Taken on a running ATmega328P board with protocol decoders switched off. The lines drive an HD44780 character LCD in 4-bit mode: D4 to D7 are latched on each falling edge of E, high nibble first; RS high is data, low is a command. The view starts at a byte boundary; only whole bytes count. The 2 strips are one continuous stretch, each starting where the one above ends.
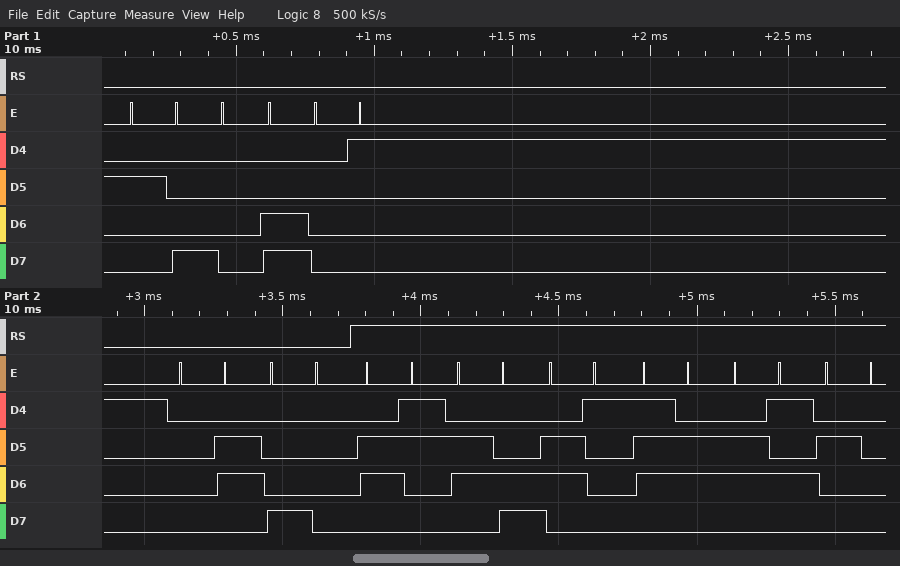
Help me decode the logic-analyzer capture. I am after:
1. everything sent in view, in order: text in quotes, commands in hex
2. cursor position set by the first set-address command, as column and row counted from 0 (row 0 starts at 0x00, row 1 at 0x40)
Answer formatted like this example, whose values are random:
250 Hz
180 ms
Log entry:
0x28 0x0C 0x01 0x06 0x80 "clave "
column 0, row 0
